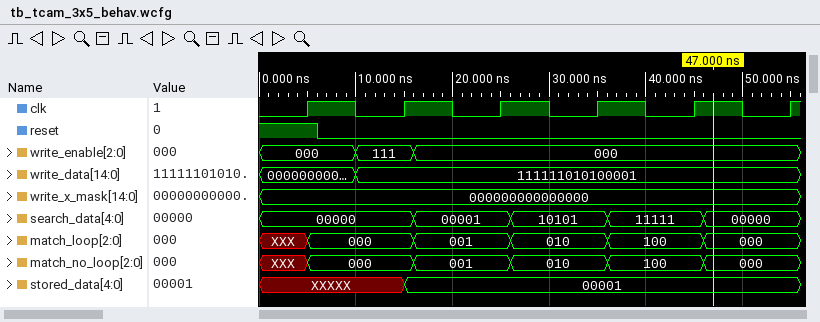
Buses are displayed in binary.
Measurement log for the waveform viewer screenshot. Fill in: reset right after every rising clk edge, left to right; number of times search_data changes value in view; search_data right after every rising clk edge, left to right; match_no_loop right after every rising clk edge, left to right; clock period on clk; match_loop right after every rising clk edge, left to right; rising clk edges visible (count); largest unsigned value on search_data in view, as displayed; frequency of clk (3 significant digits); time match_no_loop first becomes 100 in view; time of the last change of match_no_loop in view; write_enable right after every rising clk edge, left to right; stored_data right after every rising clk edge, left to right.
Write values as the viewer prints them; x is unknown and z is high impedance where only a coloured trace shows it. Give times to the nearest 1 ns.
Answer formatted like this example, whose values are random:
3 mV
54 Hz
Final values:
1 0 0 0 0 0
4
00000, 00000, 00001, 10101, 11111, 00000
000, 000, 001, 010, 100, 000
10 ns
000, 000, 001, 010, 100, 000
6
11111
100 MHz
36 ns
46 ns
000, 111, 000, 000, 000, 000
XXXXX, 00001, 00001, 00001, 00001, 00001
